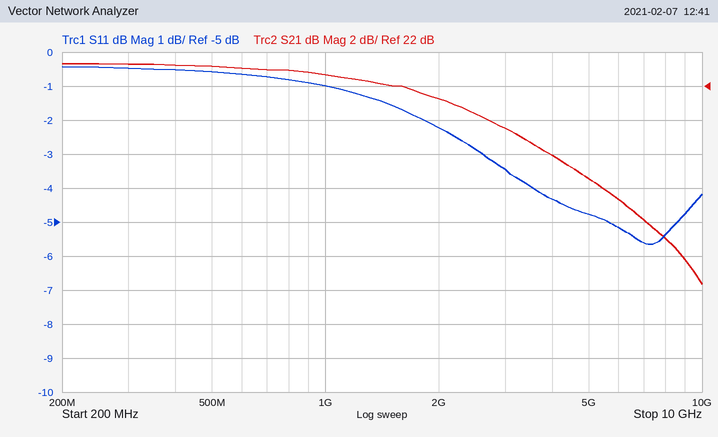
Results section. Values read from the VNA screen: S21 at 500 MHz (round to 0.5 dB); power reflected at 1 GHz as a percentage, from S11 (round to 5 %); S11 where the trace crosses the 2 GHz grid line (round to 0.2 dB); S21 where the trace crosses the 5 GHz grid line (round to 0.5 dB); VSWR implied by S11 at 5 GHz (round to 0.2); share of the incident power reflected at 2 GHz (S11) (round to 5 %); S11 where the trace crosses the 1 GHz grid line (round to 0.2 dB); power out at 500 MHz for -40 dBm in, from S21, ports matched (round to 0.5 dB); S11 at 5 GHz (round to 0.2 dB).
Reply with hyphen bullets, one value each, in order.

- 23.0 dB
- 80 %
- -2.2 dB
- 16.5 dB
- 3.8
- 60 %
- -1.0 dB
- -17.0 dBm
- -4.8 dB
